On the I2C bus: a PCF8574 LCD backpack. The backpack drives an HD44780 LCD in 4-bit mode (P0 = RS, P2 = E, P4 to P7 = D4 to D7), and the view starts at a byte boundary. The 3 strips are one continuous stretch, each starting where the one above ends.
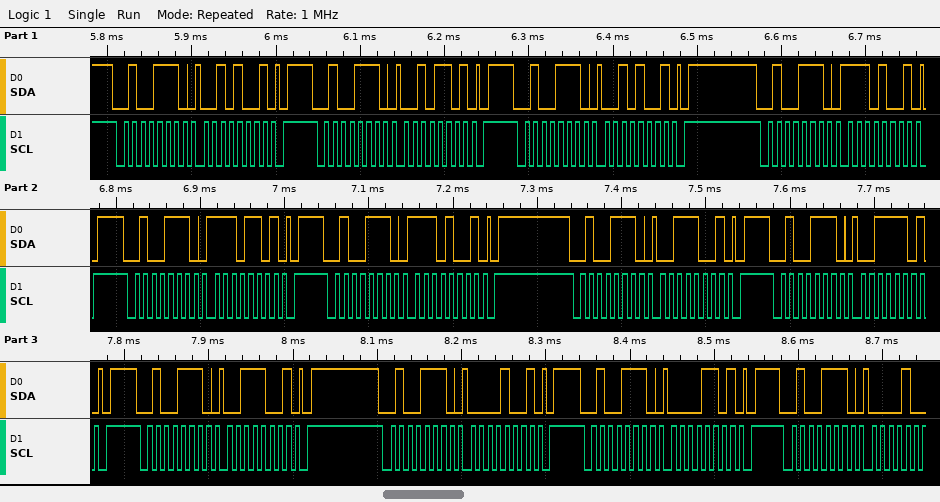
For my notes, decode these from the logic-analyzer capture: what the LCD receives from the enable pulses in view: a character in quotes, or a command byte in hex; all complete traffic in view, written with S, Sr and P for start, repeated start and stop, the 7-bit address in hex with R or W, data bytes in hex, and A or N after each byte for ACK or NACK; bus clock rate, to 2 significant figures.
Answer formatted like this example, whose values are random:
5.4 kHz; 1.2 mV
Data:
'.'; S 27W A 29 A P S 27W A 2D A P S 27W A 29 A P S 27W A E9 A P S 27W A ED A P S 27W A E9 A P S 27W A 39 A P S 27W A 3D A P S 27W A 39 A P S 27W A 09 A P S 27W A 0D A P S 27W A; 100 kHz
